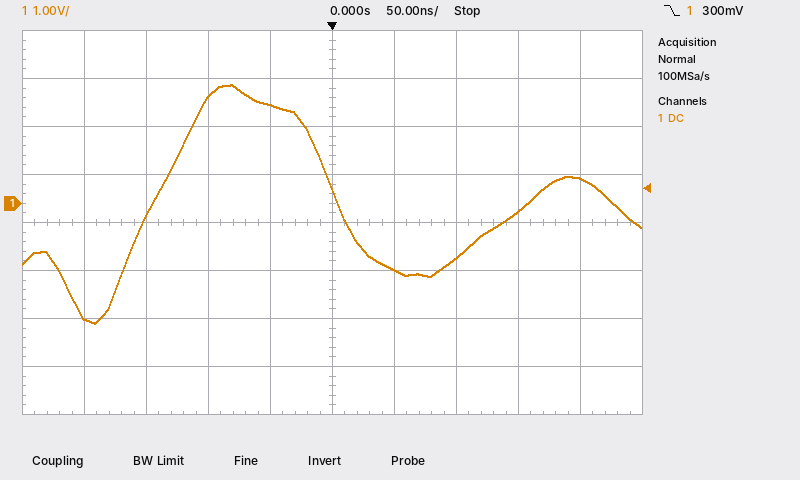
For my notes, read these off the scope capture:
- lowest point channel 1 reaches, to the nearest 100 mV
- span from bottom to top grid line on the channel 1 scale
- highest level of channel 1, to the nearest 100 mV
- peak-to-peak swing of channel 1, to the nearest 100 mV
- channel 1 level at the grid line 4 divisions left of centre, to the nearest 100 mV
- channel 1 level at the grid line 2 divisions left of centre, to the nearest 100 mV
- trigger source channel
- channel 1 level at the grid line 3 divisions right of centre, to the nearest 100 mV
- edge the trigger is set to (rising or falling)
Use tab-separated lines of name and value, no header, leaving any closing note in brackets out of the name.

lowest point channel 1 reaches, to the nearest 100 mV	-2.5 V
span from bottom to top grid line on the channel 1 scale	8 V
highest level of channel 1, to the nearest 100 mV	2.5 V
peak-to-peak swing of channel 1, to the nearest 100 mV	5.0 V
channel 1 level at the grid line 4 divisions left of centre, to the nearest 100 mV	-2.4 V
channel 1 level at the grid line 2 divisions left of centre, to the nearest 100 mV	2.2 V
trigger source channel	channel 1
channel 1 level at the grid line 3 divisions right of centre, to the nearest 100 mV	-200 mV
edge the trigger is set to	falling
